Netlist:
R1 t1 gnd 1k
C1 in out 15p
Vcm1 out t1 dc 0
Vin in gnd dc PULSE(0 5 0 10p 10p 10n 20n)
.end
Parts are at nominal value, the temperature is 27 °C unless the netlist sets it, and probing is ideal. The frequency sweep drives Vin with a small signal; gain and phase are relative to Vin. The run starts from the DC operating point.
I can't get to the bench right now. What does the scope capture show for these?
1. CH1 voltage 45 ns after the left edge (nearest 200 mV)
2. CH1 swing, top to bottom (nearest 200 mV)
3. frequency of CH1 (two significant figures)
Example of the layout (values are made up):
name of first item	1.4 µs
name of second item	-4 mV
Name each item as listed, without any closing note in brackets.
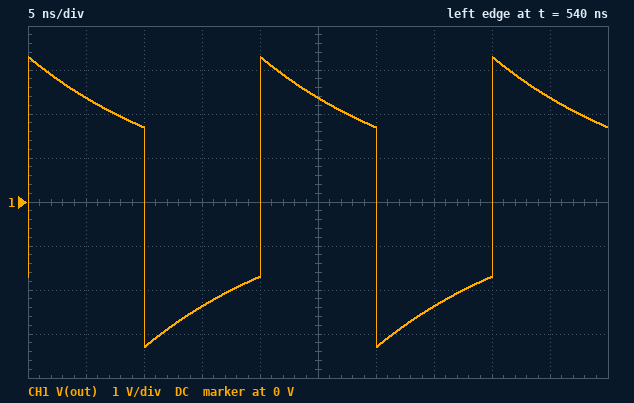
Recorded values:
CH1 voltage 45 ns after the left edge	2.4 V
CH1 swing, top to bottom	6.6 V
frequency of CH1	50 MHz
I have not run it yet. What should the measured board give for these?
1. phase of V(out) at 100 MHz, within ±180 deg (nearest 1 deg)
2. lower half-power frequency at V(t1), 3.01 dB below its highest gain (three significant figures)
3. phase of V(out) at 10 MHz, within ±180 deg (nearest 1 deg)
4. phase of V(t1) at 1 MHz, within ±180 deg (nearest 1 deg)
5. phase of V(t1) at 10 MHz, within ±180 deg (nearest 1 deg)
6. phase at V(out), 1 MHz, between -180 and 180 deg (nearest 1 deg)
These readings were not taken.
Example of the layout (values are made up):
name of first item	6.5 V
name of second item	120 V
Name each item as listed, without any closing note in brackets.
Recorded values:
phase of V(out) at 100 MHz, within ±180 deg	6 deg
lower half-power frequency at V(t1), 3.01 dB below its highest gain	10.6 MHz
phase of V(out) at 10 MHz, within ±180 deg	47 deg
phase of V(t1) at 1 MHz, within ±180 deg	85 deg
phase of V(t1) at 10 MHz, within ±180 deg	47 deg
phase at V(out), 1 MHz, between -180 and 180 deg	85 deg
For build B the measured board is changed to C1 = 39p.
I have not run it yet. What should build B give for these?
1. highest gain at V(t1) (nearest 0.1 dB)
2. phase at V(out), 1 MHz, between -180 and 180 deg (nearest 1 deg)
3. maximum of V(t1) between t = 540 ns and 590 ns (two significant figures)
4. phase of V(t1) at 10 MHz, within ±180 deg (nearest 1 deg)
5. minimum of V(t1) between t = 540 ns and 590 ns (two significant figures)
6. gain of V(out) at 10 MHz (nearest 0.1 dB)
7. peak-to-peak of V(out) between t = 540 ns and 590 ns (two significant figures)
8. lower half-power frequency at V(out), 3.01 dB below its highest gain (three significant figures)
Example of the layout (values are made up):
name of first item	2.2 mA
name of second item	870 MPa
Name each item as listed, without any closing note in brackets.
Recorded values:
highest gain at V(t1)	0 dB
phase at V(out), 1 MHz, between -180 and 180 deg	76 deg
maximum of V(t1) between t = 540 ns and 590 ns	2.8 V
phase of V(t1) at 10 MHz, within ±180 deg	22 deg
minimum of V(t1) between t = 540 ns and 590 ns	-2.8 V
gain of V(out) at 10 MHz	-0.7 dB
peak-to-peak of V(out) between t = 540 ns and 590 ns	5.6 V
lower half-power frequency at V(out), 3.01 dB below its highest gain	4.08 MHz
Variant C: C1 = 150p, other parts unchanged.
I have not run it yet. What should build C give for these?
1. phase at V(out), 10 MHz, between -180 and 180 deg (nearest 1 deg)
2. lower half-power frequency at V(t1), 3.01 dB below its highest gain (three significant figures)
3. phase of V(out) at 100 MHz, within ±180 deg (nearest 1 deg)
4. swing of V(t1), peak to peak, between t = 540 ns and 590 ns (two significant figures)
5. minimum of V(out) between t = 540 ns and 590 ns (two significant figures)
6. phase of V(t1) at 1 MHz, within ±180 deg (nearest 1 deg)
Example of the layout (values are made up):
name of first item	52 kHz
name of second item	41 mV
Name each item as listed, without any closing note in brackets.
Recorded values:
phase at V(out), 10 MHz, between -180 and 180 deg	6 deg
lower half-power frequency at V(t1), 3.01 dB below its highest gain	1.06 MHz
phase of V(out) at 100 MHz, within ±180 deg	1 deg
swing of V(t1), peak to peak, between t = 540 ns and 590 ns	5.2 V
minimum of V(out) between t = 540 ns and 590 ns	-2.5 V
phase of V(t1) at 1 MHz, within ±180 deg	47 deg
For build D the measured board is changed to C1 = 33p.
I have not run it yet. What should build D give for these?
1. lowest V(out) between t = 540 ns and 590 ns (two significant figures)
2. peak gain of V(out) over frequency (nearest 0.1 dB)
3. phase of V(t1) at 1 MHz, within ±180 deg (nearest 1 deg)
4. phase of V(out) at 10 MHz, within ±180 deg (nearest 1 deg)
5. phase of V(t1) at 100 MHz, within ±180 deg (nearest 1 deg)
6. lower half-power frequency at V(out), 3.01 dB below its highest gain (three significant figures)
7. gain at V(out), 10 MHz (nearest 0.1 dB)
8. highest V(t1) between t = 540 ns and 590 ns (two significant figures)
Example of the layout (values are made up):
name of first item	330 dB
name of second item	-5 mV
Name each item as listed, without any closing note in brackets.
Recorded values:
lowest V(out) between t = 540 ns and 590 ns	-2.9 V
peak gain of V(out) over frequency	0 dB
phase of V(t1) at 1 MHz, within ±180 deg	78 deg
phase of V(out) at 10 MHz, within ±180 deg	26 deg
phase of V(t1) at 100 MHz, within ±180 deg	3 deg
lower half-power frequency at V(out), 3.01 dB below its highest gain	4.82 MHz
gain at V(out), 10 MHz	-0.9 dB
highest V(t1) between t = 540 ns and 590 ns	2.9 V
